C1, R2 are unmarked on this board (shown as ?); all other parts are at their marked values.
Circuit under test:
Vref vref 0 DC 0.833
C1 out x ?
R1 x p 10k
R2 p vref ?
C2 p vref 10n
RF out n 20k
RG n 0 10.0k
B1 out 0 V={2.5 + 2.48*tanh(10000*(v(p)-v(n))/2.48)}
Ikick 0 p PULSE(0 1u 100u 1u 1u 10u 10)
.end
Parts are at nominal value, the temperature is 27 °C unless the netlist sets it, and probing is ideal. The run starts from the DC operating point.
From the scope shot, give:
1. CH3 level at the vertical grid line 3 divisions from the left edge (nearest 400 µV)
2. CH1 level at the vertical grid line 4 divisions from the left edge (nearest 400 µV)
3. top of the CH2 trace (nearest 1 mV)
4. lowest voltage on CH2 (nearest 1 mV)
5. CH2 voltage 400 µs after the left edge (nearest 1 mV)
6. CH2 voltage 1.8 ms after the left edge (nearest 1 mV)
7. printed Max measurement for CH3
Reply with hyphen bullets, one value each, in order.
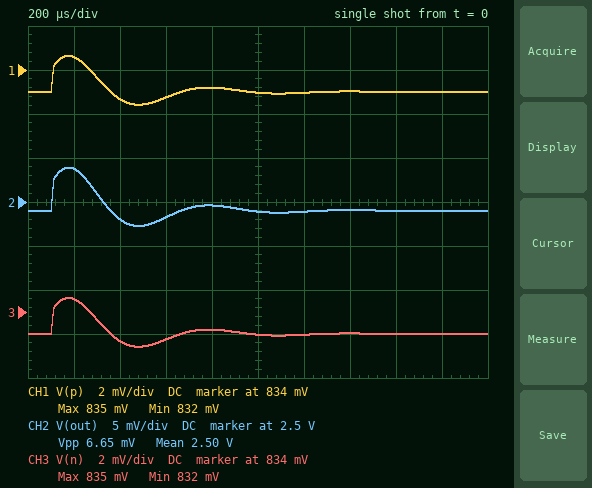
- 832.8 mV
- 833.2 mV
- 2.504 V
- 2.497 V
- 2.498 V
- 2.499 V
- 835 mV
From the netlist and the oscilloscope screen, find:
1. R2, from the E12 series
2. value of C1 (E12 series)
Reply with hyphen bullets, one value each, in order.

- 18 kΩ
- 4.7 nF
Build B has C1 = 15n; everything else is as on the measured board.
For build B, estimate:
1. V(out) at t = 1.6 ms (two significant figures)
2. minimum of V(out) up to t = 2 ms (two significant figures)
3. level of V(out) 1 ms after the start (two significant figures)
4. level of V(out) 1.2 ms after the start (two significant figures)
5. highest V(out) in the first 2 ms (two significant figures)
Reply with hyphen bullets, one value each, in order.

- 4.9 V
- 130 mV
- 2.2 V
- 2.1 V
- 5.0 V
